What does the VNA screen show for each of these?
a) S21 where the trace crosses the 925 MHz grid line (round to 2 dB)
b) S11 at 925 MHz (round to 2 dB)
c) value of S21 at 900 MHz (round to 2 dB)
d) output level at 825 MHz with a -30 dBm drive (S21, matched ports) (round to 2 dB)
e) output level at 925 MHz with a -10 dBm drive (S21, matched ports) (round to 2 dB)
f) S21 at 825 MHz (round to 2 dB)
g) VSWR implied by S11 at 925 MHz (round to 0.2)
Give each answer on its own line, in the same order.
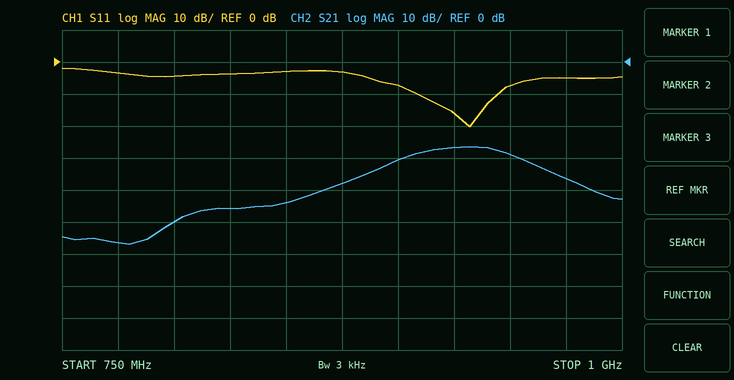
-26 dB
-16 dB
-30 dB
-76 dBm
-36 dBm
-46 dB
1.4
